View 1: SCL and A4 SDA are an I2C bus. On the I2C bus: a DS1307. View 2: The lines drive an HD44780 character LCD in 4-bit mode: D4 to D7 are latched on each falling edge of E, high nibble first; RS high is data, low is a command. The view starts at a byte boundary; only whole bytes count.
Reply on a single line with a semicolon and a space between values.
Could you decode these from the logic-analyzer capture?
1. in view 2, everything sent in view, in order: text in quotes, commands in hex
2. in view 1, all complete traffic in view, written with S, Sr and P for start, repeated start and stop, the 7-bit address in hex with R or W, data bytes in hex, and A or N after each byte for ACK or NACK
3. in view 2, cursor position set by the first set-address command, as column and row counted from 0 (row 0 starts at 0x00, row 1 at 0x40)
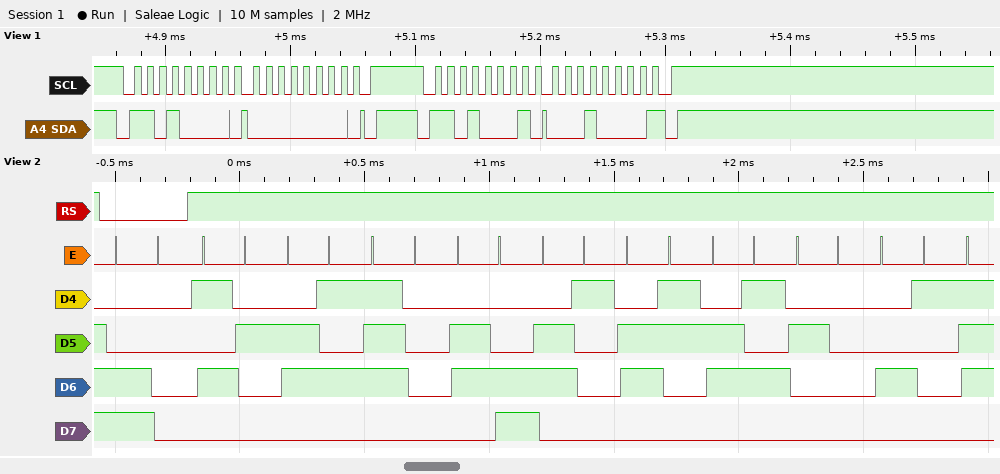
0xC0 "Replace A"; S 68W A 00 A P S 68R A 10 N P; column 0, row 1
